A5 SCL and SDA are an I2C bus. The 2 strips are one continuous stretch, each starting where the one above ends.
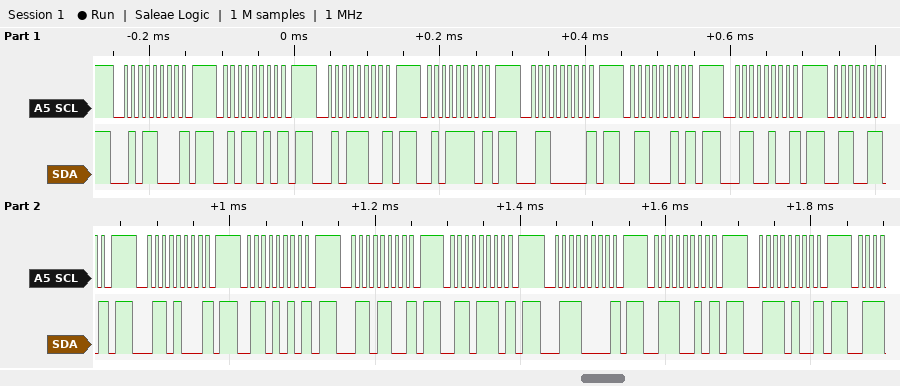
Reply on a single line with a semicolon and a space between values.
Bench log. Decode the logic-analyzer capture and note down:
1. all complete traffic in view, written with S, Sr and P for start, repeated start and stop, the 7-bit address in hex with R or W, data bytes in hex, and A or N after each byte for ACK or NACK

S 2CW N P S 2DW N P S 2EW N P S 2FW N P S 30W N P S 31W N P S 32W N P S 33W N P S 34W N P S 35W N P S 36W N P S 37W N P S 38W N P S 39W N P S 3AW N P
